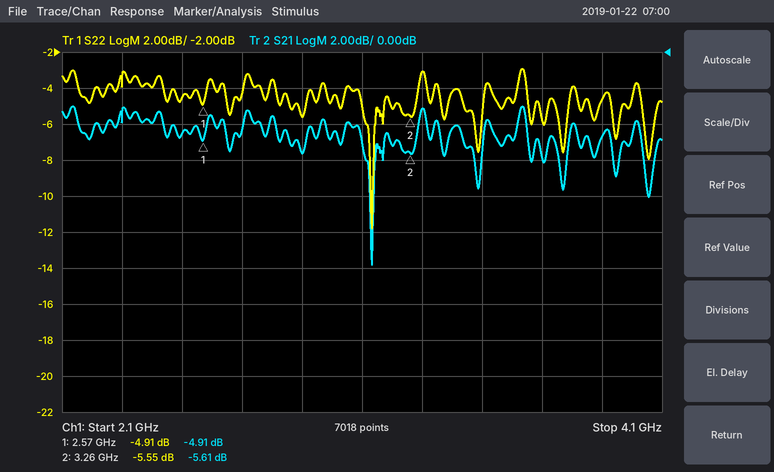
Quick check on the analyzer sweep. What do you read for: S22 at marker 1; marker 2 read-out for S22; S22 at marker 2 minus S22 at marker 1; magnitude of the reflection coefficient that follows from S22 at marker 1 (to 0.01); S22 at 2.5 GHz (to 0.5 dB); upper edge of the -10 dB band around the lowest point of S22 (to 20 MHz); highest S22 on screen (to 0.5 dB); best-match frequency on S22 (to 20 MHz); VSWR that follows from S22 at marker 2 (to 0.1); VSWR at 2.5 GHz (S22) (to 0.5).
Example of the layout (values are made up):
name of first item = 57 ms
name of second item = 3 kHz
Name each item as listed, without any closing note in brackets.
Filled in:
S22 at marker 1 = -4.91 dB
marker 2 read-out for S22 = -5.55 dB
S22 at marker 2 minus S22 at marker 1 = -0.64 dB
magnitude of the reflection coefficient that follows from S22 at marker 1 = 0.57
S22 at 2.5 GHz = -4.5 dB
upper edge of the -10 dB band around the lowest point of S22 = 3.14 GHz
highest S22 on screen = -3.0 dB
best-match frequency on S22 = 3.14 GHz
VSWR that follows from S22 at marker 2 = 3.2
VSWR at 2.5 GHz (S22) = 4.0
